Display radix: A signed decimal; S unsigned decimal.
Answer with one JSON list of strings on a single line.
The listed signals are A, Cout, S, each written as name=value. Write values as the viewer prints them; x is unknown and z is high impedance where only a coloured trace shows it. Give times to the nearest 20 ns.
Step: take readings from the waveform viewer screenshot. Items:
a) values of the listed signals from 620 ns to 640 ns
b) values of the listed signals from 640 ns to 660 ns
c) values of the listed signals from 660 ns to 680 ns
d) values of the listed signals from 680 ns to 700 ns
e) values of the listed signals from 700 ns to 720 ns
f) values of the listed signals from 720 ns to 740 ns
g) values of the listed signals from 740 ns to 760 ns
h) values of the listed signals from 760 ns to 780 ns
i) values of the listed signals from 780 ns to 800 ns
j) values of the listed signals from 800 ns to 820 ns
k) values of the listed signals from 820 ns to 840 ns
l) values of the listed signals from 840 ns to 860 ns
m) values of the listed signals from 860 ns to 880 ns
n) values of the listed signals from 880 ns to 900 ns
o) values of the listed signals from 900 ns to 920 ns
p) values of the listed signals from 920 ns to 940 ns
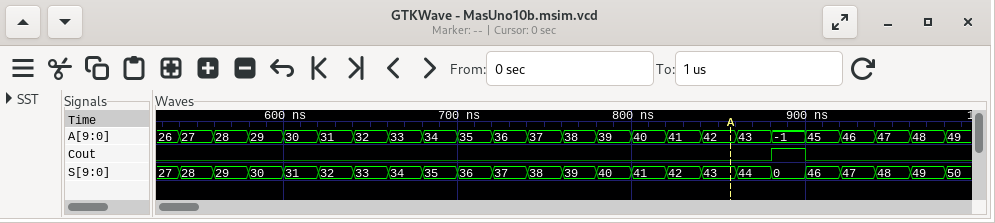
["A=31, Cout=0, S=32", "A=32, Cout=0, S=33", "A=33, Cout=0, S=34", "A=34, Cout=0, S=35", "A=35, Cout=0, S=36", "A=36, Cout=0, S=37", "A=37, Cout=0, S=38", "A=38, Cout=0, S=39", "A=39, Cout=0, S=40", "A=40, Cout=0, S=41", "A=41, Cout=0, S=42", "A=42, Cout=0, S=43", "A=43, Cout=0, S=44", "A=-1, Cout=1, S=0", "A=45, Cout=0, S=46", "A=46, Cout=0, S=47"]
